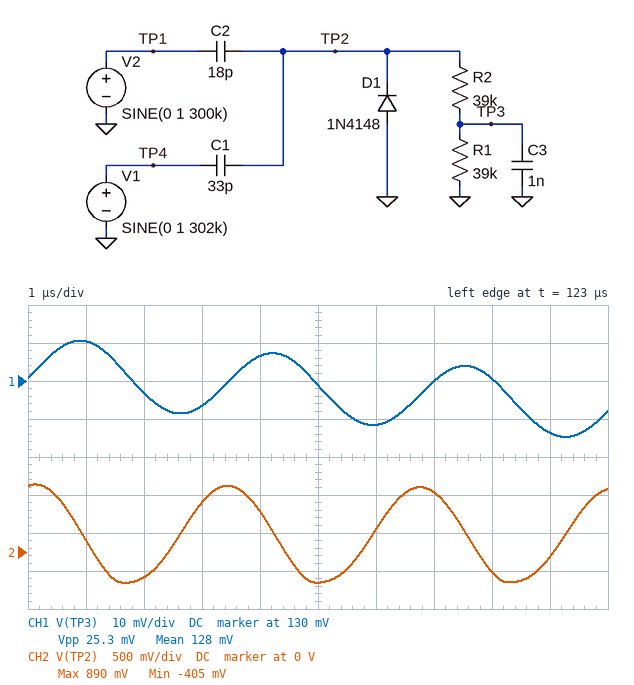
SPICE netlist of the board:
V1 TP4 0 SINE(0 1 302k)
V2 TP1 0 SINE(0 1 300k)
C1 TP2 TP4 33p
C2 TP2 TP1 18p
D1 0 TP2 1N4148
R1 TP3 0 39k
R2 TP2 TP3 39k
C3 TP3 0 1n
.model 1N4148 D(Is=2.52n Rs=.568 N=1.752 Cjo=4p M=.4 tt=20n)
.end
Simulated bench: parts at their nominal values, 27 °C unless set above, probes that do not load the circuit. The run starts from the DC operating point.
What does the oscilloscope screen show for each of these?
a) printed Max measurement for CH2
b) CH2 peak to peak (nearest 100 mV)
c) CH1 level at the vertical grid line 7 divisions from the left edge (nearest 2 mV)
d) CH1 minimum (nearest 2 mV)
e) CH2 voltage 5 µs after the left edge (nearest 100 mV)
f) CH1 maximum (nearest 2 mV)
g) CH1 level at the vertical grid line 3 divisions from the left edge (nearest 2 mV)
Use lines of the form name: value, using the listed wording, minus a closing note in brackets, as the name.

printed Max measurement for CH2: 890 mV
CH2 peak to peak: 1.3 V
CH1 level at the vertical grid line 7 divisions from the left edge: 130 mV
CH1 minimum: 116 mV
CH2 voltage 5 µs after the left edge: -400 mV
CH1 maximum: 140 mV
CH1 level at the vertical grid line 3 divisions from the left edge: 124 mV
